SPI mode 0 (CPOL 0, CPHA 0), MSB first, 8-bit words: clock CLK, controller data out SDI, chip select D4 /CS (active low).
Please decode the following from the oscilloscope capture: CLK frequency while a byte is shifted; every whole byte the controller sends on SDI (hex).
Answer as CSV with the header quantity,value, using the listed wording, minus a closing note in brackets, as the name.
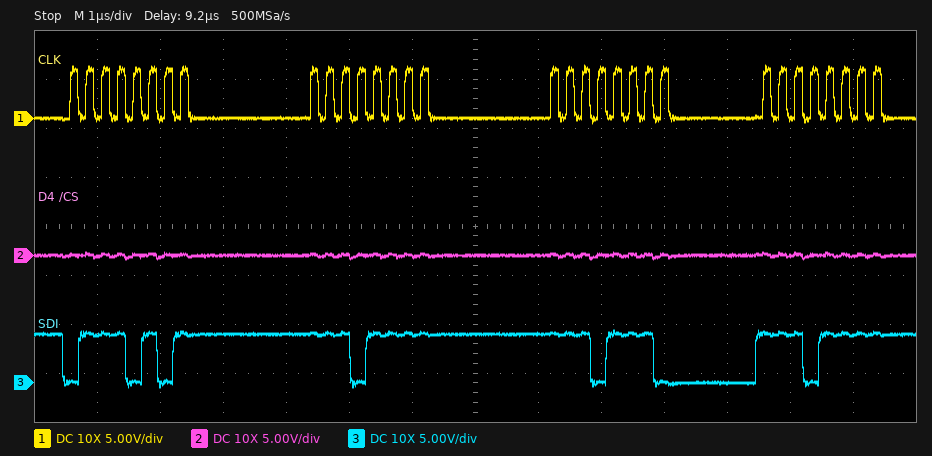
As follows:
quantity,value
CLK frequency while a byte is shifted,4 MHz
every whole byte the controller sends on SDI,75 EF EE EF
